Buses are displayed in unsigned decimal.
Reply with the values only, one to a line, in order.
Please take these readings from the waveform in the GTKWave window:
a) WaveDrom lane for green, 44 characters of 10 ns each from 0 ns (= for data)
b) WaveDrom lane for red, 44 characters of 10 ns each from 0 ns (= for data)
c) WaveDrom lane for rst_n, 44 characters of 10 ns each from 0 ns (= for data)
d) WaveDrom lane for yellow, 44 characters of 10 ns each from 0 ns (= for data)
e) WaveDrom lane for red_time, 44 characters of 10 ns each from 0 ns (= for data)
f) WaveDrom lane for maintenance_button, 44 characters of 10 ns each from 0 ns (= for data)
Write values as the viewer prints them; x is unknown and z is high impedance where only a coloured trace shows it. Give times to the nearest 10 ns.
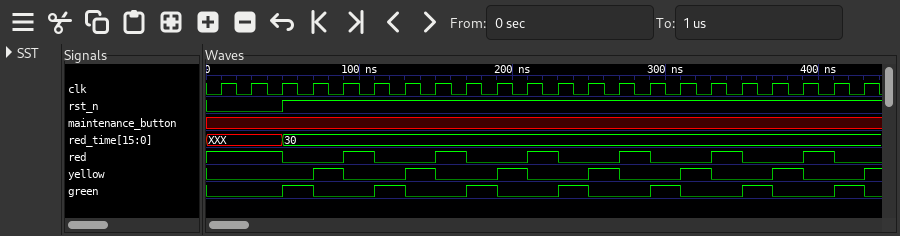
{name: 'green', wave: '0....1.0...1.0...1.0...1.0...1.0...1.0...1.0'}
{name: 'red', wave: '1....0...1.0...1.0...1.0...1.0...1.0...1.0..'}
{name: 'rst_n', wave: '0....1......................................'}
{name: 'yellow', wave: '0......1.0...1.0...1.0...1.0...1.0...1.0...1'}
{name: 'red_time', wave: 'x....=......................................', data: '30'}
{name: 'maintenance_button', wave: 'x...........................................'}
